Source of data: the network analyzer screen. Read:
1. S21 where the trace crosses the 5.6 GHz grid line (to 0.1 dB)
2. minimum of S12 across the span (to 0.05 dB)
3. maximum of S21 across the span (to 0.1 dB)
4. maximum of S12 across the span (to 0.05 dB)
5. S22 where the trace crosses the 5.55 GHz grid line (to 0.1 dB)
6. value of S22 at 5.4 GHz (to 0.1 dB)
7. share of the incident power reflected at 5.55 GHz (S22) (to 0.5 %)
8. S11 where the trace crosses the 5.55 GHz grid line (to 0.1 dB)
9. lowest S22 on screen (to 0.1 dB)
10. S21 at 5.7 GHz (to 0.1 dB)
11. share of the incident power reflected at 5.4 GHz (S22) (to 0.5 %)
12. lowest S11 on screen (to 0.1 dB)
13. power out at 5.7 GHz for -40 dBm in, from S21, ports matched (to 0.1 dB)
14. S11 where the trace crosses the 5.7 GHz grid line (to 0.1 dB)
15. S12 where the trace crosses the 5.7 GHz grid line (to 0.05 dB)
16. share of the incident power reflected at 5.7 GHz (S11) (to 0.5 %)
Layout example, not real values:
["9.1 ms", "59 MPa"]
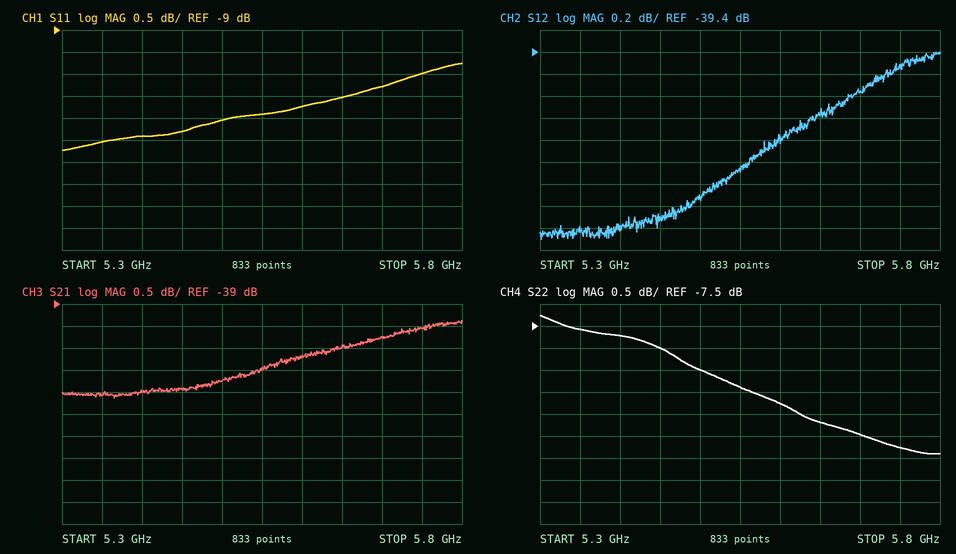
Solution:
["-40.2 dB", "-41.10 dB", "-39.4 dB", "-39.40 dB", "-8.9 dB", "-7.7 dB", "13.0 %", "-10.9 dB", "-10.4 dB", "-39.8 dB", "17.0 %", "-11.7 dB", "-79.8 dBm", "-10.3 dB", "-39.75 dB", "9.5 %"]
